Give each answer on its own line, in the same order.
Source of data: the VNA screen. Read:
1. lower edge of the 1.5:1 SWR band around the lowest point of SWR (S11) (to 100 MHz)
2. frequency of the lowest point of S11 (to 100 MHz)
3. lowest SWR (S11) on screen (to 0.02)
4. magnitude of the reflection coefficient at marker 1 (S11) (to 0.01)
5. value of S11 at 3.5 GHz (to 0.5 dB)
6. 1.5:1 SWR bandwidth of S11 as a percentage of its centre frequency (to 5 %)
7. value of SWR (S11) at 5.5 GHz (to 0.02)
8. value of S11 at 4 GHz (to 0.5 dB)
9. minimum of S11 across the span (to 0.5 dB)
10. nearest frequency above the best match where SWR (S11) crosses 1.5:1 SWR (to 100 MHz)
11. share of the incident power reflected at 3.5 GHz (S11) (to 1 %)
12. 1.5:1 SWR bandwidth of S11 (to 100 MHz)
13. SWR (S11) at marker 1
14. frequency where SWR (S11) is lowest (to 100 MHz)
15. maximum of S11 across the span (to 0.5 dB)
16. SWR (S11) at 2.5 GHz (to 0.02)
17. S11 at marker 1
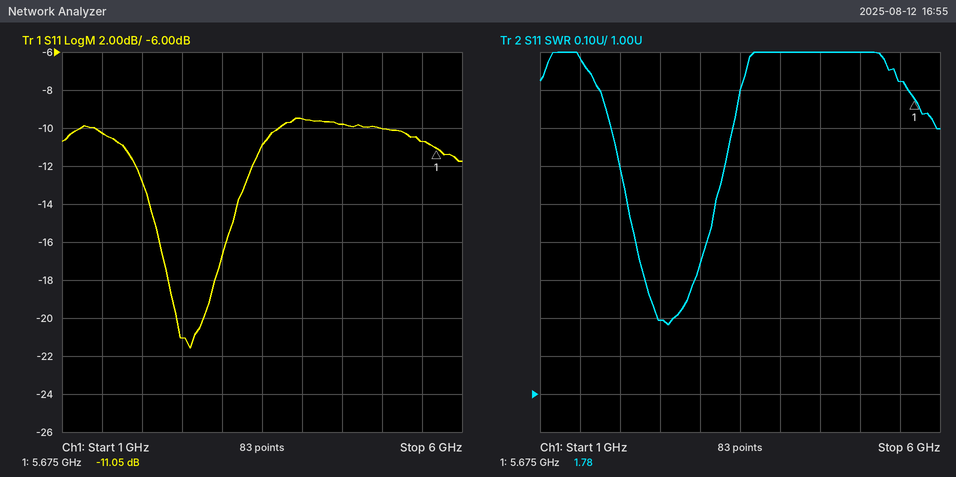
2.1 GHz
2.6 GHz
1.18
0.28
-11.0 dB
40 %
1.82
-9.5 dB
-21.5 dB
3.2 GHz
8 %
1.1 GHz
1.78
2.6 GHz
-9.5 dB
1.20
-11.05 dB
